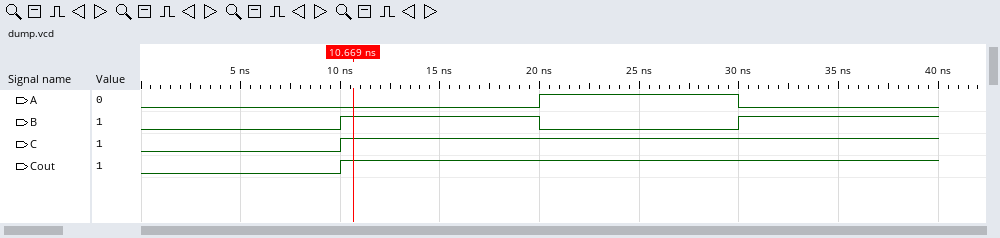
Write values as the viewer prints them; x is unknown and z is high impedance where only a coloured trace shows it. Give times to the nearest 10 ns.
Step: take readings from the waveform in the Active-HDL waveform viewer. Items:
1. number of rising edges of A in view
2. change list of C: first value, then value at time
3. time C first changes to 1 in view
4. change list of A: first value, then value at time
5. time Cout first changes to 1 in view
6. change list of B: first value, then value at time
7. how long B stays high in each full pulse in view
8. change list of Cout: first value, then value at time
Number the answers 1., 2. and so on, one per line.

1. 1
2. 0, 1 at 10 ns
3. 10 ns
4. 0, 1 at 20 ns, 0 at 30 ns
5. 10 ns
6. 0, 1 at 10 ns, 0 at 20 ns, 1 at 30 ns
7. 10 ns
8. 0, 1 at 10 ns
